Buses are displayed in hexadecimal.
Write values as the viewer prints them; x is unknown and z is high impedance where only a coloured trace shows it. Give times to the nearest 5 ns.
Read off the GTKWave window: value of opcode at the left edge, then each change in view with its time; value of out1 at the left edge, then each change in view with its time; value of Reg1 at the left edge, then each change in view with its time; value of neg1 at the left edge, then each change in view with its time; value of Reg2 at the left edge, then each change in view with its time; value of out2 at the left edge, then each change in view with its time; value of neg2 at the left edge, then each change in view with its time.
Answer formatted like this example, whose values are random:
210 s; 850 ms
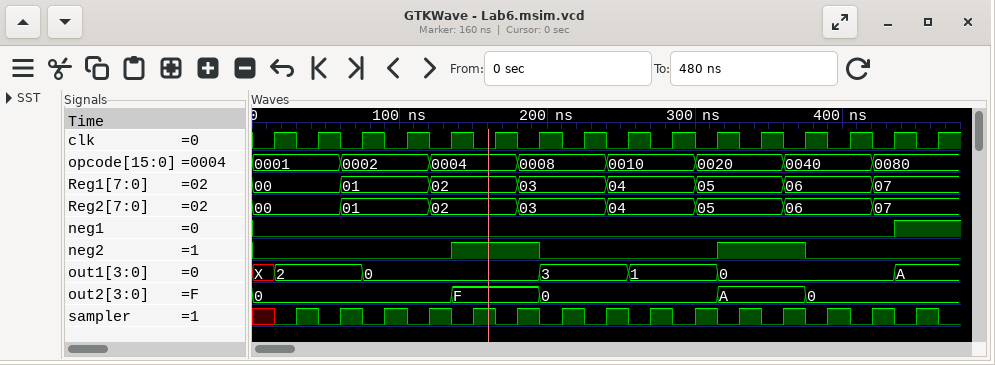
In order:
0001, 0002 at 60 ns, 0004 at 120 ns, 0008 at 180 ns, 0010 at 240 ns, 0020 at 300 ns, 0040 at 360 ns, 0080 at 420 ns; X, 2 at 15 ns, 0 at 75 ns, 3 at 195 ns, 1 at 255 ns, 0 at 315 ns, A at 435 ns; 00, 01 at 60 ns, 02 at 120 ns, 03 at 180 ns, 04 at 240 ns, 05 at 300 ns, 06 at 360 ns, 07 at 420 ns; 0, 1 at 435 ns; 00, 01 at 60 ns, 02 at 120 ns, 03 at 180 ns, 04 at 240 ns, 05 at 300 ns, 06 at 360 ns, 07 at 420 ns; 0, F at 135 ns, 0 at 195 ns, A at 315 ns, 0 at 375 ns; 0, 1 at 135 ns, 0 at 195 ns, 1 at 315 ns, 0 at 375 ns
